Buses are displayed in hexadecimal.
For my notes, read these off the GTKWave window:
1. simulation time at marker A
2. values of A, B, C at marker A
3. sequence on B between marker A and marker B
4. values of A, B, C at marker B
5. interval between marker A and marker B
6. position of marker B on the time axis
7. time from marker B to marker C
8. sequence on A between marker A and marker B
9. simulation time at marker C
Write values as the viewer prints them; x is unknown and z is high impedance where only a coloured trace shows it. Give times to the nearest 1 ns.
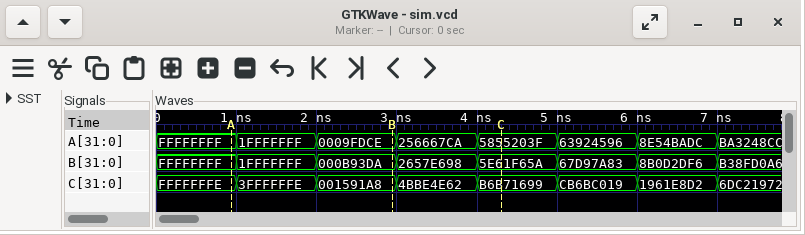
1 ns
A=FFFFFFFF, B=FFFFFFFF, C=FFFFFFFE
FFFFFFFF, 1FFFFFFF, 000B93DA
A=0009FDCE, B=000B93DA, C=001591A8
2 ns
3 ns
1 ns
FFFFFFFF, 1FFFFFFF, 0009FDCE
4 ns
